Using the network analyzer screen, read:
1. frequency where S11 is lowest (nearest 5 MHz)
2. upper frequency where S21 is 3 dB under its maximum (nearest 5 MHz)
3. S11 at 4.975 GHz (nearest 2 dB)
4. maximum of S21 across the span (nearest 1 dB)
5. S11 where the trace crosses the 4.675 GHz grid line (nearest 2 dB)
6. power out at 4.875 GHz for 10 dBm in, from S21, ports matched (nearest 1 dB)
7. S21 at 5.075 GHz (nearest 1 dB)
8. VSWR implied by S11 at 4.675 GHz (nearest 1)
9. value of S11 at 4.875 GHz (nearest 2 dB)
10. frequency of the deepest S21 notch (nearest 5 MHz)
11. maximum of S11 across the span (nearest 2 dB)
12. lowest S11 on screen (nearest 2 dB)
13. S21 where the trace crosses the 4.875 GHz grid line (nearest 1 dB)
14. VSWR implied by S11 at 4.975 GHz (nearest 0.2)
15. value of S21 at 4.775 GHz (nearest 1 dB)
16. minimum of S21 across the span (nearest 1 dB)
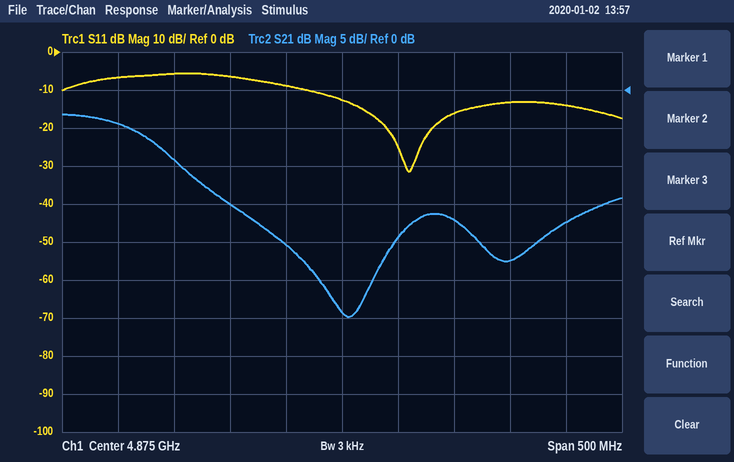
4.935 GHz
4.700 GHz
-16 dB
-3 dB
-6 dB
-19 dBm
-17 dB
3
-12 dB
4.880 GHz
-6 dB
-32 dB
-29 dB
1.4
-15 dB
-30 dB
